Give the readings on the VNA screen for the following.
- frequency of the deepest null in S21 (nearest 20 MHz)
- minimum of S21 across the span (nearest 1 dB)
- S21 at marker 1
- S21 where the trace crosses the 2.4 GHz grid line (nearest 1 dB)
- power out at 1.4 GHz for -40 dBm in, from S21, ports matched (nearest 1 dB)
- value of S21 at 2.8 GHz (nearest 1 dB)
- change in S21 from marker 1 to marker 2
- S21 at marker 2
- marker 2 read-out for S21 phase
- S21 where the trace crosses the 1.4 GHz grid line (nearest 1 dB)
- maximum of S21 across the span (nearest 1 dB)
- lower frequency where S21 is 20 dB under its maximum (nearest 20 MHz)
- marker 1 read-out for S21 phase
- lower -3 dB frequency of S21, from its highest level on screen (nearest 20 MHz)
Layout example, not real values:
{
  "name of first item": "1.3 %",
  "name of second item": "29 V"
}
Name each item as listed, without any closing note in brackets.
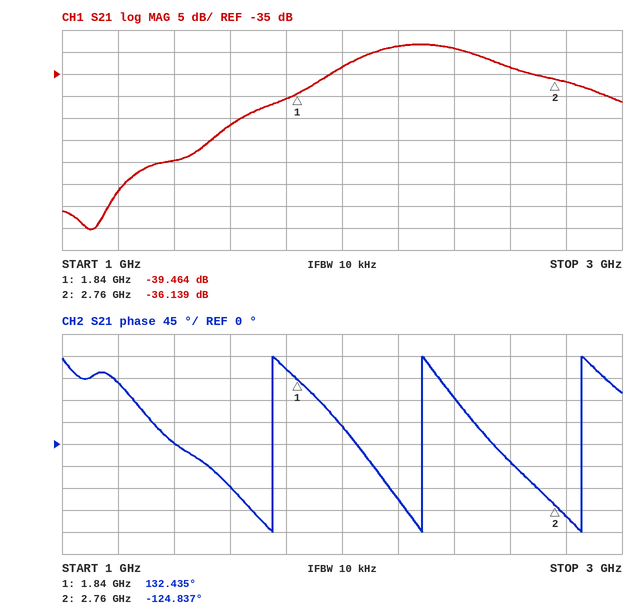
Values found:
{
  "frequency of the deepest null in S21": "1.10 GHz",
  "minimum of S21 across the span": "-70 dB",
  "S21 at marker 1": "-39.464 dB",
  "S21 where the trace crosses the 2.4 GHz grid line": "-29 dB",
  "power out at 1.4 GHz for -40 dBm in, from S21, ports matched": "-95 dBm",
  "value of S21 at 2.8 GHz": "-37 dB",
  "change in S21 from marker 1 to marker 2": "3.325 dB",
  "S21 at marker 2": "-36.139 dB",
  "marker 2 read-out for S21 phase": "-124.837°",
  "S21 where the trace crosses the 1.4 GHz grid line": "-55 dB",
  "maximum of S21 across the span": "-28 dB",
  "lower frequency where S21 is 20 dB under its maximum": "1.56 GHz",
  "marker 1 read-out for S21 phase": "132.435°",
  "lower -3 dB frequency of S21, from its highest level on screen": "2.06 GHz"
}
